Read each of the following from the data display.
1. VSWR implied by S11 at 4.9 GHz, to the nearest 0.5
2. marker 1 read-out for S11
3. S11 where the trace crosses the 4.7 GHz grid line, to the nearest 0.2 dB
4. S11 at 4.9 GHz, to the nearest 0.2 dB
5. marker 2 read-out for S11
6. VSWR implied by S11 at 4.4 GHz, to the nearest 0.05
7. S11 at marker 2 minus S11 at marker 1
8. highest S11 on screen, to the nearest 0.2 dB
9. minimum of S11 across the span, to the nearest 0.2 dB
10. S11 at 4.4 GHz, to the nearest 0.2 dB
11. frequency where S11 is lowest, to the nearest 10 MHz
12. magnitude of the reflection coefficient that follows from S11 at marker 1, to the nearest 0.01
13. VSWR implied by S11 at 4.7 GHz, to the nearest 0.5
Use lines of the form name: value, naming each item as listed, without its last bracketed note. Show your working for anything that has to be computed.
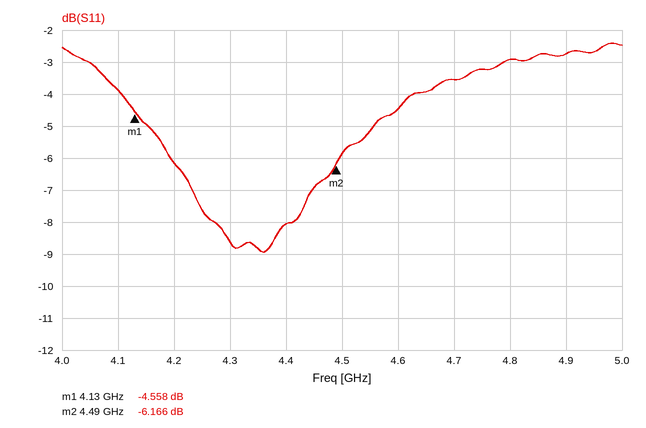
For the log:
VSWR implied by S11 at 4.9 GHz, to the nearest 0.5: |Γ| = 10^(-2.8/20) = 0.7244; VSWR = (1 + 0.7244)/(1 − 0.7244) ≈ 6.26, so 6.5 to the nearest 0.5
marker 1 read-out for S11: -4.558 dB
S11 where the trace crosses the 4.7 GHz grid line, to the nearest 0.2 dB: -3.6 dB
S11 at 4.9 GHz, to the nearest 0.2 dB: -2.8 dB
marker 2 read-out for S11: -6.166 dB
VSWR implied by S11 at 4.4 GHz, to the nearest 0.05: |Γ| = 10^(-8/20) = 0.3981; VSWR = (1 + 0.3981)/(1 − 0.3981) ≈ 2.32, so 2.30 to the nearest 0.05
S11 at marker 2 minus S11 at marker 1: -6.166 − (-4.558) = -1.608 dB
highest S11 on screen, to the nearest 0.2 dB: -2.4 dB
minimum of S11 across the span, to the nearest 0.2 dB: -9.0 dB
S11 at 4.4 GHz, to the nearest 0.2 dB: -8.0 dB
frequency where S11 is lowest, to the nearest 10 MHz: 4.36 GHz
magnitude of the reflection coefficient that follows from S11 at marker 1, to the nearest 0.01: 10^(-4.558/20) ≈ 0.59
VSWR implied by S11 at 4.7 GHz, to the nearest 0.5: |Γ| = 10^(-3.6/20) = 0.6607; VSWR = (1 + 0.6607)/(1 − 0.6607) ≈ 4.89, so 5.0 to the nearest 0.5
